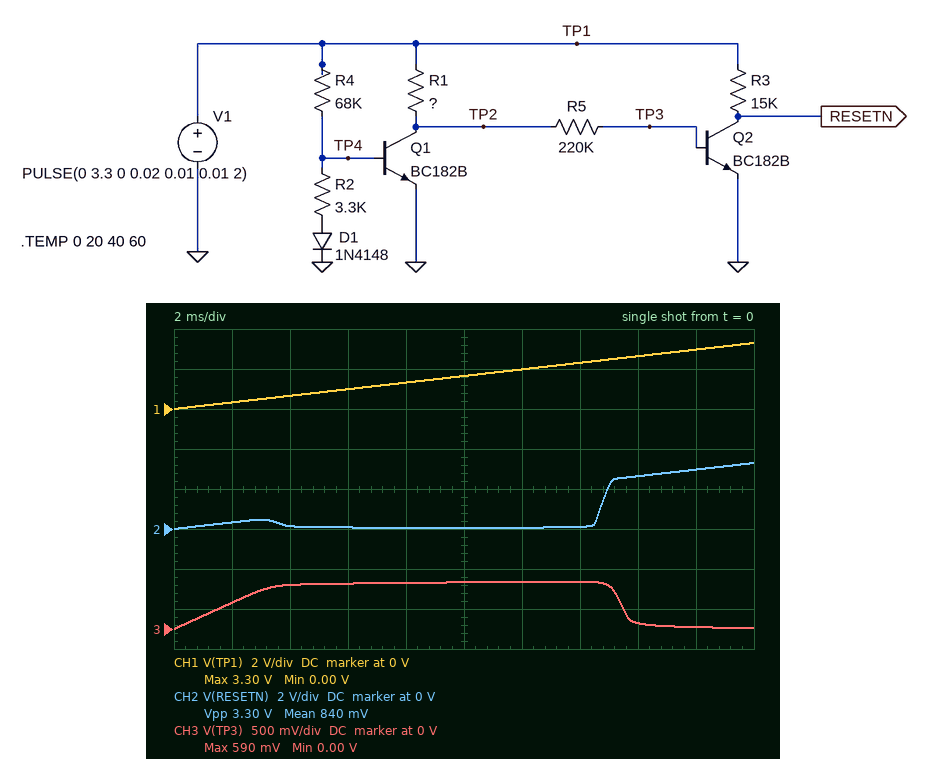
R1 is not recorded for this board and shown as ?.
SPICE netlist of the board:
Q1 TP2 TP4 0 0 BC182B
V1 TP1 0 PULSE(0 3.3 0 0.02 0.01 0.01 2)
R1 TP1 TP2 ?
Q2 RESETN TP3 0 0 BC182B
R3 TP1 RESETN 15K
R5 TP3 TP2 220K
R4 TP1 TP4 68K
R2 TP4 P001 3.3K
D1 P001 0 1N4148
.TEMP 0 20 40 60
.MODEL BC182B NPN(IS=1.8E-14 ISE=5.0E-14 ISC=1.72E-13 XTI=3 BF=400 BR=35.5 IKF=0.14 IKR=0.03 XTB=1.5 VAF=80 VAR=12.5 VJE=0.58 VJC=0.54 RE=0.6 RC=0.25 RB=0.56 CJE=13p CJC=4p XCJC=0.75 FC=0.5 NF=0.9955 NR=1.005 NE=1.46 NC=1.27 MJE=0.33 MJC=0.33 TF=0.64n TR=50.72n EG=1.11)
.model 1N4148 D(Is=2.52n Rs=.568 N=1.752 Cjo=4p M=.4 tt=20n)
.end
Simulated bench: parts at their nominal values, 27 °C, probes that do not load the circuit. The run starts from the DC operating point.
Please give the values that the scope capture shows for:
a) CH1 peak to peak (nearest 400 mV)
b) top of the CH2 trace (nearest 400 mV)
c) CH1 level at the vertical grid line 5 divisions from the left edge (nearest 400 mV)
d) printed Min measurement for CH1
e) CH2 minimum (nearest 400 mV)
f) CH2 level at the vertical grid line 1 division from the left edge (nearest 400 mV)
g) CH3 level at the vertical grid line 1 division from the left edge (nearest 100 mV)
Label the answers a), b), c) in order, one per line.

a) 3.2 V
b) 3.2 V
c) 1.6 V
d) 0.00 V
e) 0 V
f) 400 mV
g) 300 mV
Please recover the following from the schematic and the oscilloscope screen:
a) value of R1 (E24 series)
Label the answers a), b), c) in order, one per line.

a) 200 kΩ
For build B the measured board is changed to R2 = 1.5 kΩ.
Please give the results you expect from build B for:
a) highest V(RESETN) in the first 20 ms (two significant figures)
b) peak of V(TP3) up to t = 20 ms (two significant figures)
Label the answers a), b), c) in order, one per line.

a) 460 mV
b) 600 mV
